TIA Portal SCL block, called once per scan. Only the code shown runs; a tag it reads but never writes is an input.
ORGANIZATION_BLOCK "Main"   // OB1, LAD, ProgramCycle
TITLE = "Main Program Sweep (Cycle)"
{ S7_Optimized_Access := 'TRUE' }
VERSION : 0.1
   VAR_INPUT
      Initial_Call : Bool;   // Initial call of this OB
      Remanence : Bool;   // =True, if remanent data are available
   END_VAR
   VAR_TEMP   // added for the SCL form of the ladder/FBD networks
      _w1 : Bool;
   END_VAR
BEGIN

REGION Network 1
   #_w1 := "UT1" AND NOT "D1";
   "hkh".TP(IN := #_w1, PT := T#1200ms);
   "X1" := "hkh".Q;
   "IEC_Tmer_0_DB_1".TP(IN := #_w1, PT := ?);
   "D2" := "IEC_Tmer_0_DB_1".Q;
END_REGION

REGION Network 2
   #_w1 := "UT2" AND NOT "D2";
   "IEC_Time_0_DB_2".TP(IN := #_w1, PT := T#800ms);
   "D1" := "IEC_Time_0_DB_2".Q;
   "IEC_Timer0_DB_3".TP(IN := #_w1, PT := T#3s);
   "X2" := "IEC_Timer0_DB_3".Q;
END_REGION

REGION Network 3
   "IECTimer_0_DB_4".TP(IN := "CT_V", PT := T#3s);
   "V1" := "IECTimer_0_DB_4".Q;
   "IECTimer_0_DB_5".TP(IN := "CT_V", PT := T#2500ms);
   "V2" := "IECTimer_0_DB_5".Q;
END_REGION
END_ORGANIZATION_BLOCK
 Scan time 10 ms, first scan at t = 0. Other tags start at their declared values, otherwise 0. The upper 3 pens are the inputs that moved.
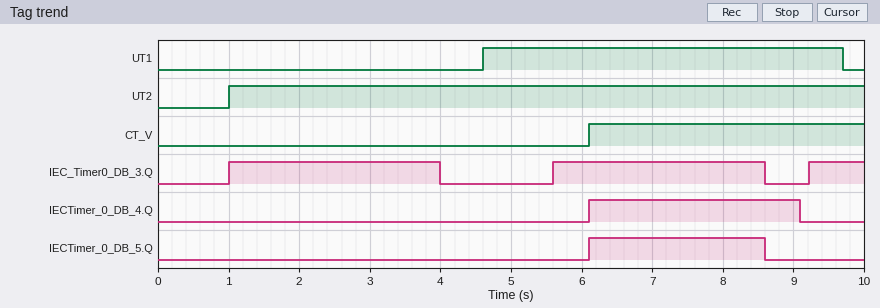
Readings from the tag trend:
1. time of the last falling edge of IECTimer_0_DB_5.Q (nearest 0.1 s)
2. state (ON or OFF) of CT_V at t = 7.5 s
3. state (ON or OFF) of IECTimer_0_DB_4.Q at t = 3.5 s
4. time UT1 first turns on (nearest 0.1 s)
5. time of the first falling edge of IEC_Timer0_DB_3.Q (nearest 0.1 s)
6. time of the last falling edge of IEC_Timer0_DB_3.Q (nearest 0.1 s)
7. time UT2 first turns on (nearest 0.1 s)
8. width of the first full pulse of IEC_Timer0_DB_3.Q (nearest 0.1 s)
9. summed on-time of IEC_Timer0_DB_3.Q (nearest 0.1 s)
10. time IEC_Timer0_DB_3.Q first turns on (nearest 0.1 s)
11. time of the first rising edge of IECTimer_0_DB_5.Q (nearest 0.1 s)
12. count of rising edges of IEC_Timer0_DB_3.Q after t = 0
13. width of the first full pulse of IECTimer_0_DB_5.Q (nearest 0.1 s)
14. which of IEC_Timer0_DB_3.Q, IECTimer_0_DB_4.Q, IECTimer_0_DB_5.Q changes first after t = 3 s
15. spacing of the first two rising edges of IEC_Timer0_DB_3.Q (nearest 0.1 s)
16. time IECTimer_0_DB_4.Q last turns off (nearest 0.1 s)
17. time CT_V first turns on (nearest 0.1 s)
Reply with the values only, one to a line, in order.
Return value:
8.6 s
ON
OFF
4.6 s
4.0 s
8.6 s
1.0 s
3.0 s
6.8 s
1.0 s
6.1 s
3
2.5 s
IEC_Timer0_DB_3.Q
4.6 s
9.1 s
6.1 s
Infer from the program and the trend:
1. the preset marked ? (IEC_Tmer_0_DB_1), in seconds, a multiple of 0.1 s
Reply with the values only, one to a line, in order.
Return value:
1.0 s
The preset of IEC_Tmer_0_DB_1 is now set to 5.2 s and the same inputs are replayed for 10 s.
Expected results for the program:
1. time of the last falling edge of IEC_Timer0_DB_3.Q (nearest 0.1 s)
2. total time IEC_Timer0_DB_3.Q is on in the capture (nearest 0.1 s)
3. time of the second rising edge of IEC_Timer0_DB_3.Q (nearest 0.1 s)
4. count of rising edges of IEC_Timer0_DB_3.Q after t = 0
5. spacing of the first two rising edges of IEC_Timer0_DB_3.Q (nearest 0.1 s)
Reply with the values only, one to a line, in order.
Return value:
4.0 s
3.2 s
9.8 s
2
8.8 s
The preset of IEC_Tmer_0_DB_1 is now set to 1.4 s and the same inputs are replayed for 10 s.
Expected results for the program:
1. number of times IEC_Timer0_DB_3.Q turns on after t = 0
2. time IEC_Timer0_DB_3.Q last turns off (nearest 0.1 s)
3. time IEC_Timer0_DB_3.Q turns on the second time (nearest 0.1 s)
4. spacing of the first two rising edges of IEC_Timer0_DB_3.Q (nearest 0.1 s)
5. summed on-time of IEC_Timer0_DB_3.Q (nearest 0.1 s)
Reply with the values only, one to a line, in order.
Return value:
2
9.0 s
6.0 s
5.0 s
6.0 s
